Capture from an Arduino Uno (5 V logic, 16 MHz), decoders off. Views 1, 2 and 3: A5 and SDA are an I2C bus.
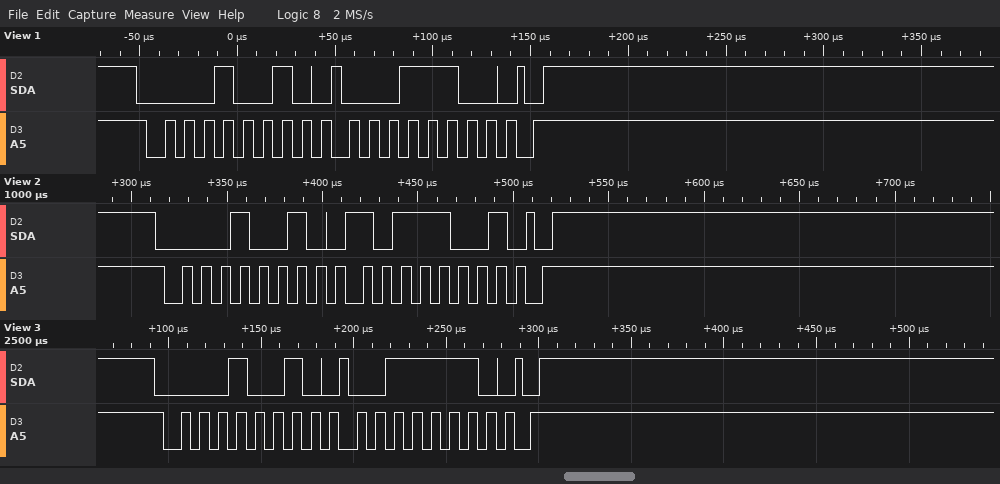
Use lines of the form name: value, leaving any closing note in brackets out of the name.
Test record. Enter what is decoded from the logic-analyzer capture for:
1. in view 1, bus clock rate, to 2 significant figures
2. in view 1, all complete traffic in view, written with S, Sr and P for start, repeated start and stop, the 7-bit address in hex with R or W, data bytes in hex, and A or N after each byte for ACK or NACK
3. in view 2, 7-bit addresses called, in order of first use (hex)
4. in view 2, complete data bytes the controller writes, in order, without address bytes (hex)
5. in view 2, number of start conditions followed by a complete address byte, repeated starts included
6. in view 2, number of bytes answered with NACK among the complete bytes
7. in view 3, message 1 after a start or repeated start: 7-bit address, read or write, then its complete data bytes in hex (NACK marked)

in view 1, bus clock rate, to 2 significant figures: 100 kHz
in view 1, all complete traffic in view, written with S, Sr and P for start, repeated start and stop, the 7-bit address in hex with R or W, data bytes in hex, and A or N after each byte for ACK or NACK: S 09W A 1C A P
in view 2, 7-bit addresses called, in order of first use: 0x09
in view 2, complete data bytes the controller writes, in order, without address bytes: B9
in view 2, number of start conditions followed by a complete address byte, repeated starts included: 1
in view 2, number of bytes answered with NACK among the complete bytes: 0
in view 3, message 1 after a start or repeated start: 7-bit address, read or write, then its complete data bytes in hex: 0x09 write: 3E
